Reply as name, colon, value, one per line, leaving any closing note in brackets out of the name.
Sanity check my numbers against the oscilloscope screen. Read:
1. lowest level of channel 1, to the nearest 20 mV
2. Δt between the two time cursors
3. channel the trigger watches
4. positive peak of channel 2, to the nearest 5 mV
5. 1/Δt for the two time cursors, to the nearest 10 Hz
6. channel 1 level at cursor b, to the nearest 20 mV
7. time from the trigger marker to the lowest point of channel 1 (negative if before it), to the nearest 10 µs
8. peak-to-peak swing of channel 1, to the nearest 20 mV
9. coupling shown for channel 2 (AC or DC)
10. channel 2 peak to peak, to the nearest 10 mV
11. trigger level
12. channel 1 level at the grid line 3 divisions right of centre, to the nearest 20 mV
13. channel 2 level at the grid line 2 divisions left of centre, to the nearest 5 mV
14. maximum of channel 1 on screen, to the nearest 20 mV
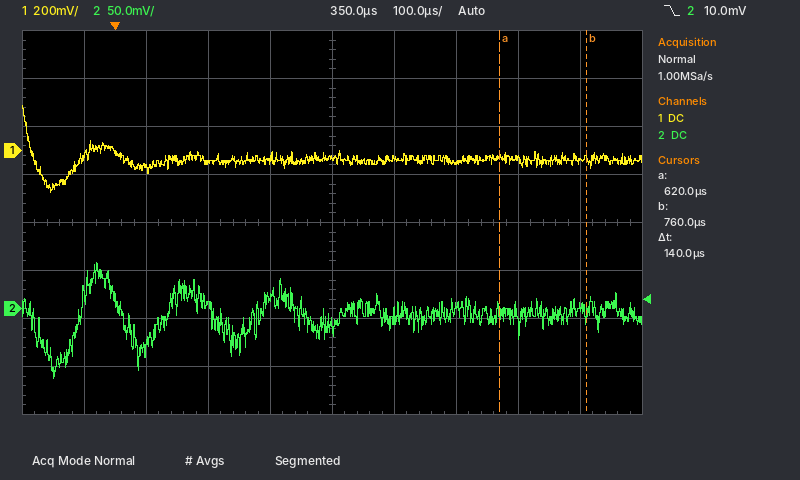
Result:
lowest level of channel 1, to the nearest 20 mV: -180 mV
Δt between the two time cursors: 140 µs
channel the trigger watches: channel 2
positive peak of channel 2, to the nearest 5 mV: 50 mV
1/Δt for the two time cursors, to the nearest 10 Hz: 7.14 kHz
channel 1 level at cursor b, to the nearest 20 mV: -40 mV
time from the trigger marker to the lowest point of channel 1 (negative if before it), to the nearest 10 µs: -100 µs
peak-to-peak swing of channel 1, to the nearest 20 mV: 360 mV
coupling shown for channel 2: DC
channel 2 peak to peak, to the nearest 10 mV: 120 mV
trigger level: 10.0 mV
channel 1 level at the grid line 3 divisions right of centre, to the nearest 20 mV: -40 mV
channel 2 level at the grid line 2 divisions left of centre, to the nearest 5 mV: 5 mV
maximum of channel 1 on screen, to the nearest 20 mV: 180 mV
